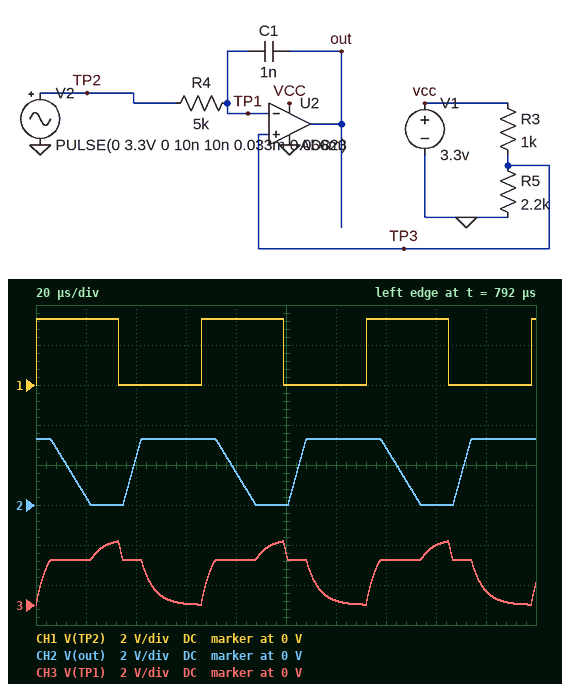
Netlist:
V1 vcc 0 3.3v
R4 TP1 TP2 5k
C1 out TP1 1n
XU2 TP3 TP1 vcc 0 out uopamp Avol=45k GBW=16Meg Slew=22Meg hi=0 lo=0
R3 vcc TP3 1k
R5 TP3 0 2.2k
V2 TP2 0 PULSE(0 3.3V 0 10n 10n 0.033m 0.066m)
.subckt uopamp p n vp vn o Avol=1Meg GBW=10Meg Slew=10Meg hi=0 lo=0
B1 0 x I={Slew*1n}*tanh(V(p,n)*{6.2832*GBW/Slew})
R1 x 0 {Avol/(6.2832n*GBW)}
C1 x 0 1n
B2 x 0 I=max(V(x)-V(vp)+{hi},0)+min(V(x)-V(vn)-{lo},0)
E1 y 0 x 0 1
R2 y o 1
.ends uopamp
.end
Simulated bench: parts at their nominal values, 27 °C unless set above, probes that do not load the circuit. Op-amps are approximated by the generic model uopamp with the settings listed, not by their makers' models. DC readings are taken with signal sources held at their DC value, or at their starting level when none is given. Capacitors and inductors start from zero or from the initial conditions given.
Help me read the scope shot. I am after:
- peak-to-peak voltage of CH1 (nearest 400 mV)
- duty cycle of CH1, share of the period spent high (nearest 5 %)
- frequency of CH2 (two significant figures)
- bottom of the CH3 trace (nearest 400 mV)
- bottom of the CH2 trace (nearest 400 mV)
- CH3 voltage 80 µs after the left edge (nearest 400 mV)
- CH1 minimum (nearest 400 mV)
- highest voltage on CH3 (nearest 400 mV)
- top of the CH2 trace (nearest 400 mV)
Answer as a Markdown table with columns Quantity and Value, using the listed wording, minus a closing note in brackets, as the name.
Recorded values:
| Quantity | Value |
|---|---|
| peak-to-peak voltage of CH1 | 3.2 V |
| duty cycle of CH1, share of the period spent high | 50 % |
| frequency of CH2 | 15 kHz |
| bottom of the CH3 trace | 0 V |
| bottom of the CH2 trace | 0 V |
| CH3 voltage 80 µs after the left edge | 2.4 V |
| CH1 minimum | 0 V |
| highest voltage on CH3 | 3.2 V |
| top of the CH2 trace | 3.2 V |
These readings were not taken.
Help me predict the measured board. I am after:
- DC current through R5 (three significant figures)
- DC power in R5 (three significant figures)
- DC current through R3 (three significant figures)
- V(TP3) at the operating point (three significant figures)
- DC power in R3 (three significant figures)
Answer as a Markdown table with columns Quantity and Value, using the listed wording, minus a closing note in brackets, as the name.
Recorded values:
| Quantity | Value |
|---|---|
| DC current through R5 | 1.03 mA |
| DC power in R5 | 2.34 mW |
| DC current through R3 | 1.03 mA |
| V(TP3) at the operating point | 2.27 V |
| DC power in R3 | 1.06 mW |
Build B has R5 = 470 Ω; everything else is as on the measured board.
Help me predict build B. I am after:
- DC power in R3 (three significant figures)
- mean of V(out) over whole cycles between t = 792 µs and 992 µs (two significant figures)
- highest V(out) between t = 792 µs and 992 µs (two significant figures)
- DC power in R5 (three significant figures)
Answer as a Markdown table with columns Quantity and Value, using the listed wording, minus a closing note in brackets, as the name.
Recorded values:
| Quantity | Value |
|---|---|
| DC power in R3 | 5.04 mW |
| mean of V(out) over whole cycles between t = 792 µs and 992 µs | 1.2 V |
| highest V(out) between t = 792 µs and 992 µs | 3.3 V |
| DC power in R5 | 2.37 mW |
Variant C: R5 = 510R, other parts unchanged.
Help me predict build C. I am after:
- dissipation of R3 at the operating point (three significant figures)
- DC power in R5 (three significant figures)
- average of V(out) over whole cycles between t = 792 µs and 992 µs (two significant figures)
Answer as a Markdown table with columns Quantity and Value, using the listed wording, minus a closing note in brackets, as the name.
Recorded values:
| Quantity | Value |
|---|---|
| dissipation of R3 at the operating point | 4.78 mW |
| DC power in R5 | 2.44 mW |
| average of V(out) over whole cycles between t = 792 µs and 992 µs | 1.3 V |
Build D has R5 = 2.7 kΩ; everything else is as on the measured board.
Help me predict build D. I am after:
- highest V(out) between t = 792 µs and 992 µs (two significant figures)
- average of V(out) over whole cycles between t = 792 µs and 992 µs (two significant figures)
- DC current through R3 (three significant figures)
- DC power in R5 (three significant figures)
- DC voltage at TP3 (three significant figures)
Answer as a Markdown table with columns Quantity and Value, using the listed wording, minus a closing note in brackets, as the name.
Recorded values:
| Quantity | Value |
|---|---|
| highest V(out) between t = 792 µs and 992 µs | 3.3 V |
| average of V(out) over whole cycles between t = 792 µs and 992 µs | 2.2 V |
| DC current through R3 | 892 µA |
| DC power in R5 | 2.15 mW |
| DC voltage at TP3 | 2.41 V |
